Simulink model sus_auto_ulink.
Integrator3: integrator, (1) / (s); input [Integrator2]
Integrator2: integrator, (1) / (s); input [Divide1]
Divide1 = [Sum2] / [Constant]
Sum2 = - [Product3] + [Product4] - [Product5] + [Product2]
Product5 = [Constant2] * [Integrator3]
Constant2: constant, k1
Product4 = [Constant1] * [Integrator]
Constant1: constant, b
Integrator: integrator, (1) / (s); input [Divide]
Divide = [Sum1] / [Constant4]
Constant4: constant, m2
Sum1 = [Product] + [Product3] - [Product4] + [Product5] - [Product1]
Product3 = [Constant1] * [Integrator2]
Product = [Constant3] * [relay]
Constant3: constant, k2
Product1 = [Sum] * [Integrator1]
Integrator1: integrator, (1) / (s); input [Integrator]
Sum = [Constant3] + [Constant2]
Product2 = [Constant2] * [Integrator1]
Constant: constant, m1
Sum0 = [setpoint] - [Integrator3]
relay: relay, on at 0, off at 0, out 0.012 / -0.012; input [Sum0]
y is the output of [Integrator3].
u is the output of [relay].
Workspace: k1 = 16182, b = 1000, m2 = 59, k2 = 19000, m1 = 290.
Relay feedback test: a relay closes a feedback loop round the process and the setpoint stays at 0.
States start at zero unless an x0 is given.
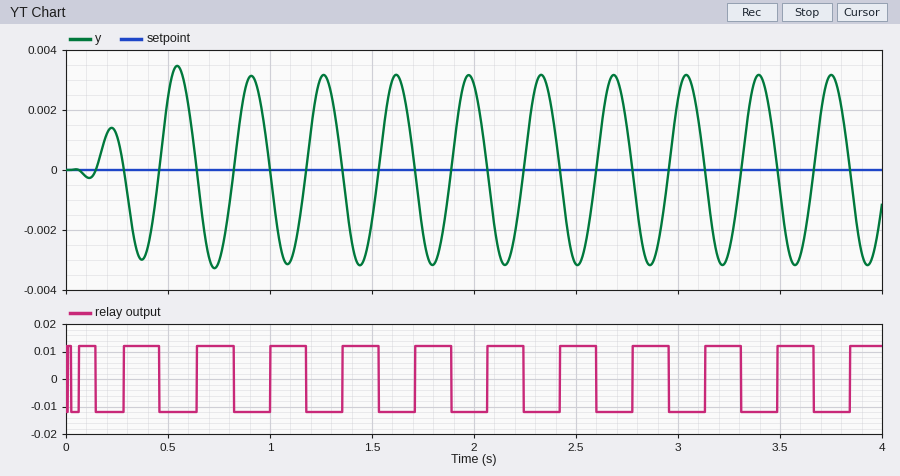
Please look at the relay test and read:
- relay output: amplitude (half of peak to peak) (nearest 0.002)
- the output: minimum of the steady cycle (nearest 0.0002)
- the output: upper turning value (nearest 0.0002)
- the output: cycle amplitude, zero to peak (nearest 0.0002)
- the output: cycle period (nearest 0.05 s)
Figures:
0.012
-0.0032
0.0032
0.0032
0.35 s
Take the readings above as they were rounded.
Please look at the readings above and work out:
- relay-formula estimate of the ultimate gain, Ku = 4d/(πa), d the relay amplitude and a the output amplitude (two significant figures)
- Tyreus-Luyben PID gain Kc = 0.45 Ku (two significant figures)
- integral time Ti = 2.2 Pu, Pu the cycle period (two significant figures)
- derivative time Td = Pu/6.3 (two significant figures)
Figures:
4.8
2.2
0.77 s
0.056 s
